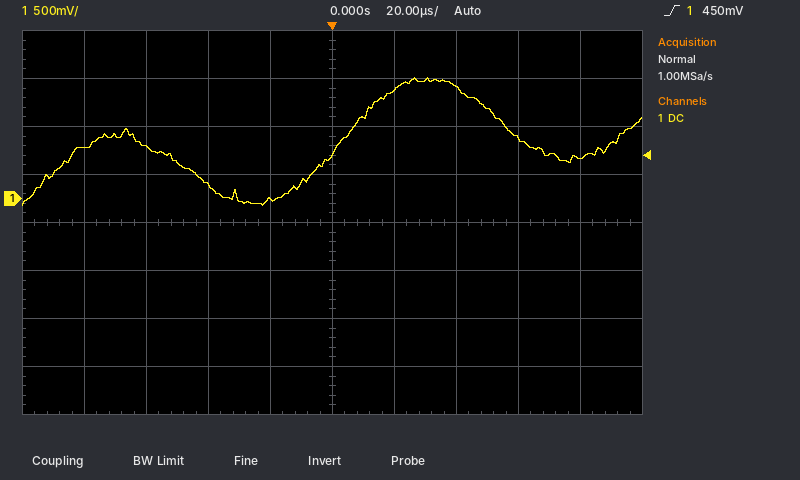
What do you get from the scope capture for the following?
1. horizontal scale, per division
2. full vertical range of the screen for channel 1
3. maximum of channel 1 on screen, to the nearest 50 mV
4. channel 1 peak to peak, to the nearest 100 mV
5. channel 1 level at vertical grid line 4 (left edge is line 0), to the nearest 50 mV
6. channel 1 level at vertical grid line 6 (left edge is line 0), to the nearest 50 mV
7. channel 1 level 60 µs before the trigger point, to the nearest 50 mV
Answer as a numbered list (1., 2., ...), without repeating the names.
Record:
1. 20 µs
2. 4 V
3. 1.25 V
4. 1.30 V
5. 0 mV
6. 1.15 V
7. 550 mV
